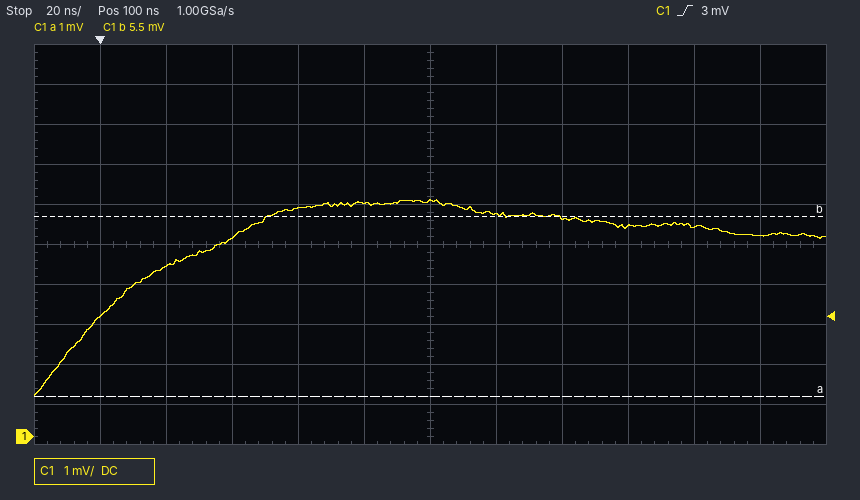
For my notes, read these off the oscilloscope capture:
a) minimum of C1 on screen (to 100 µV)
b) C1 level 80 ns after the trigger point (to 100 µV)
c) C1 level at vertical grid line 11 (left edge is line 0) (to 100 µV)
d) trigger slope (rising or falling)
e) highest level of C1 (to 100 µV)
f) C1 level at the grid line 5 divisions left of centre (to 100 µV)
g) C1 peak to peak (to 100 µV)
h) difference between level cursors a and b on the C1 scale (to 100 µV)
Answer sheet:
1.0 mV
5.8 mV
5.0 mV
rising
5.9 mV
3.0 mV
4.9 mV
4.5 mV
